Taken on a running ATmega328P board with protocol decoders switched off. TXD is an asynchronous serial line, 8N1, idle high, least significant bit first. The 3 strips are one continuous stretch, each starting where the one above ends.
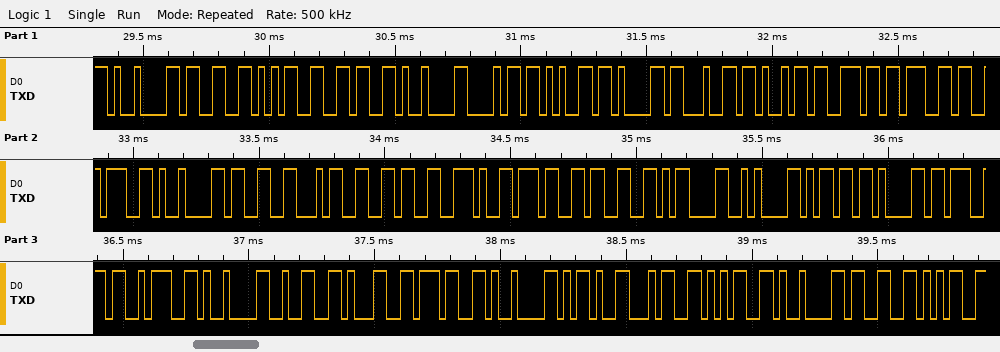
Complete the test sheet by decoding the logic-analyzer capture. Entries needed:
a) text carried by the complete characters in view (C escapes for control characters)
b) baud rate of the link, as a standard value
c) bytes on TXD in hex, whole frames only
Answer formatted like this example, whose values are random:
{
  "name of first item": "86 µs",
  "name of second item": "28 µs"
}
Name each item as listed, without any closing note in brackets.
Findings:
{
  "text carried by the complete characters in view": "\"\\t356\\theading:\\t346.73\\r\\nmag:\\t217\\t-45\\t35\"",
  "baud rate of the link, as a standard value": "38400 baud",
  "bytes on TXD in hex, whole frames only": "09 33 35 36 09 68 65 61 64 69 6E 67 3A 09 33 34 36 2E 37 33 0D 0A 6D 61 67 3A 09 32 31 37 09 2D 34 35 09 33 35"
}
